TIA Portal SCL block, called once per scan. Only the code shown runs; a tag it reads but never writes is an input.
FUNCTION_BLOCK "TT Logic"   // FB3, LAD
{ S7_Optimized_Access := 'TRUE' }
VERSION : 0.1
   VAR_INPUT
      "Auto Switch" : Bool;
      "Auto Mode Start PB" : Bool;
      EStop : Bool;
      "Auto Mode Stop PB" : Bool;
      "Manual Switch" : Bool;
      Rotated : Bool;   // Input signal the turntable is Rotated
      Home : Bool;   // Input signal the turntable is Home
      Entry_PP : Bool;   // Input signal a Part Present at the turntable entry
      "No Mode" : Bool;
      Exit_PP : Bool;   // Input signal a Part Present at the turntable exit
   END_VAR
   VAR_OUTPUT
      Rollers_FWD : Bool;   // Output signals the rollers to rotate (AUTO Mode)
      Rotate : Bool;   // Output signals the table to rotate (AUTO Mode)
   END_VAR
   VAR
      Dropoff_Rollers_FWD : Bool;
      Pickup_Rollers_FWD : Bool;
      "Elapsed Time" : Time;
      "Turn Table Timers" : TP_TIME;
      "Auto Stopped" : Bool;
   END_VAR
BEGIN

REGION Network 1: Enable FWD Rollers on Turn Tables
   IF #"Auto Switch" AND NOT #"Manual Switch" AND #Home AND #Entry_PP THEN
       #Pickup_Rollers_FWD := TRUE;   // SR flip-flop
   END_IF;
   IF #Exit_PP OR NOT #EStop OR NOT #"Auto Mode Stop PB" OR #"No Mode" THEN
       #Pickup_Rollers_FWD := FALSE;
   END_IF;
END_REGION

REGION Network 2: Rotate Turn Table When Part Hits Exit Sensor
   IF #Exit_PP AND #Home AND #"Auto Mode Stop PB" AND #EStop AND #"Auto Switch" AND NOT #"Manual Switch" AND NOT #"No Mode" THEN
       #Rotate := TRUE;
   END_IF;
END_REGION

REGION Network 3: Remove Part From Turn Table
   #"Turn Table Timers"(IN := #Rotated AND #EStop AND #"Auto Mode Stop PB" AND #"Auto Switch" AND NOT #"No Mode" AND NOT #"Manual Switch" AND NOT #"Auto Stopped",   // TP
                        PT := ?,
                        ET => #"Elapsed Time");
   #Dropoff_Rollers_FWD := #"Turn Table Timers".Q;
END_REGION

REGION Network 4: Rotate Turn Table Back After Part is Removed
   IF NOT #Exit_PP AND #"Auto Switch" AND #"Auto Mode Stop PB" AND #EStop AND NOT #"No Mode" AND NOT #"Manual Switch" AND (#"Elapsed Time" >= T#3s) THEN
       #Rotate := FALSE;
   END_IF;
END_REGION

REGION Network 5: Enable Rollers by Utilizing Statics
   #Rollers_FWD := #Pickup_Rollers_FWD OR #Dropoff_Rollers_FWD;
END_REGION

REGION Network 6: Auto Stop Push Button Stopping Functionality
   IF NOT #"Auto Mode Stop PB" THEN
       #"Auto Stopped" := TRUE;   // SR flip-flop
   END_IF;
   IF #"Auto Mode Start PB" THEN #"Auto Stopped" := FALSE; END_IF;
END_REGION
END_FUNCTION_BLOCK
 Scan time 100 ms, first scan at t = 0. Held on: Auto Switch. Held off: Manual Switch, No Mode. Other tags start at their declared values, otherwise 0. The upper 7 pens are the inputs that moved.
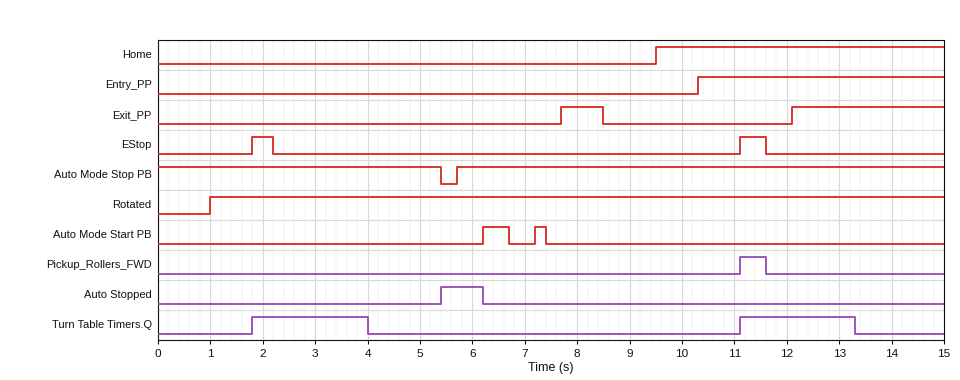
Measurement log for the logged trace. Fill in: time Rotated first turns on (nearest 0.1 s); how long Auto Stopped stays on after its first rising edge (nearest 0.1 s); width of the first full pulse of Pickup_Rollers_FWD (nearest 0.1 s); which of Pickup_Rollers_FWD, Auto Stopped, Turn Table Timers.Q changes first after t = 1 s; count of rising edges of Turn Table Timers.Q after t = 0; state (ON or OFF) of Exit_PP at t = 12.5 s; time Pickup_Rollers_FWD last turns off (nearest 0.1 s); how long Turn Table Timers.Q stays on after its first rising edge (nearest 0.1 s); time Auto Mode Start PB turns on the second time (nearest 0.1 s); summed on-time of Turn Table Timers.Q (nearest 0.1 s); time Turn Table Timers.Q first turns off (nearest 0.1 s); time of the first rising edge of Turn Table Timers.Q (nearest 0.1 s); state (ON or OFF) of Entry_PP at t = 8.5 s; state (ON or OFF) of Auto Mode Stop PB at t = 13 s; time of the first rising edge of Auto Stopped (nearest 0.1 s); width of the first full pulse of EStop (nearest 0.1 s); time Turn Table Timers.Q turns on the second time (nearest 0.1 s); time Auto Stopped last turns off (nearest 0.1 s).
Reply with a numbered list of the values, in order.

1. 1.0 s
2. 0.8 s
3. 0.5 s
4. Turn Table Timers.Q
5. 2
6. ON
7. 11.6 s
8. 2.2 s
9. 7.2 s
10. 4.4 s
11. 4.0 s
12. 1.8 s
13. OFF
14. ON
15. 5.4 s
16. 0.4 s
17. 11.1 s
18. 6.2 s
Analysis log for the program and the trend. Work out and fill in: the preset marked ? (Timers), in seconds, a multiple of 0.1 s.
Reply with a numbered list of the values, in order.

1. 2.2 s
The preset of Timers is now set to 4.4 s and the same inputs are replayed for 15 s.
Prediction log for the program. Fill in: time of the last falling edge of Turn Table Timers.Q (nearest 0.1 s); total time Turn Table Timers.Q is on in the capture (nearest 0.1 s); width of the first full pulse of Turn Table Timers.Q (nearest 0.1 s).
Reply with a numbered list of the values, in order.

1. 6.2 s
2. 8.3 s
3. 4.4 s
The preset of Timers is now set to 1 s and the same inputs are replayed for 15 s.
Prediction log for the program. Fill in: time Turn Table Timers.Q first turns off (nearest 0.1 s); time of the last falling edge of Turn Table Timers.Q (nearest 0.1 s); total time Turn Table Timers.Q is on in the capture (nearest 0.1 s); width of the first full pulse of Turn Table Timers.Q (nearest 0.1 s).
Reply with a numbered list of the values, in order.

1. 2.8 s
2. 12.1 s
3. 2.0 s
4. 1.0 s
